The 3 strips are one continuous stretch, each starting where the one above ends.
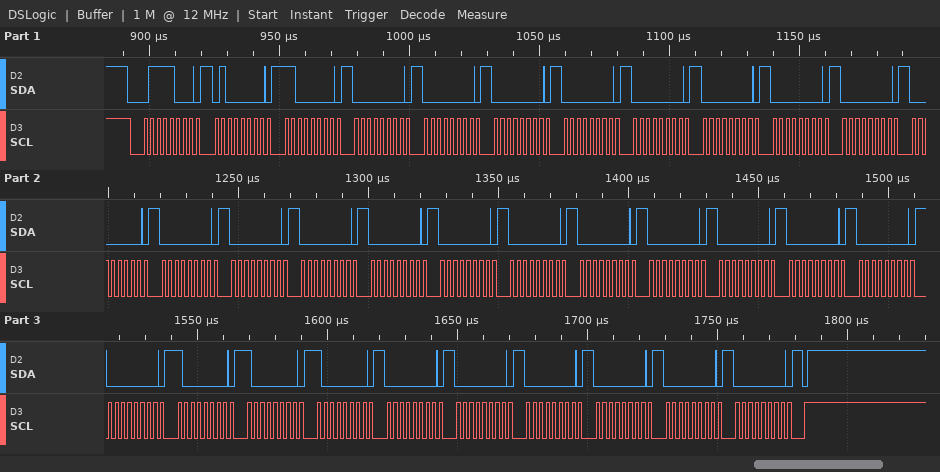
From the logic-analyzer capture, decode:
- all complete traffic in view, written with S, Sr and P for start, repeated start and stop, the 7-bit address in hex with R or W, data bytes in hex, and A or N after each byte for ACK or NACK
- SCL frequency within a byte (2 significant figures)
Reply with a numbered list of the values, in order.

1. S 3CW A 40 A C0 A 00 A 00 A 00 A 00 A 00 A 00 A 00 A 00 A 00 A 00 A 00 A 00 A 00 A 00 A 00 A 00 A 00 A 00 A 00 A 00 A 00 A 80 A 80 A 80 A 00 A 00 A 00 A 00 A 00 A 00 A P
2. 400 kHz
